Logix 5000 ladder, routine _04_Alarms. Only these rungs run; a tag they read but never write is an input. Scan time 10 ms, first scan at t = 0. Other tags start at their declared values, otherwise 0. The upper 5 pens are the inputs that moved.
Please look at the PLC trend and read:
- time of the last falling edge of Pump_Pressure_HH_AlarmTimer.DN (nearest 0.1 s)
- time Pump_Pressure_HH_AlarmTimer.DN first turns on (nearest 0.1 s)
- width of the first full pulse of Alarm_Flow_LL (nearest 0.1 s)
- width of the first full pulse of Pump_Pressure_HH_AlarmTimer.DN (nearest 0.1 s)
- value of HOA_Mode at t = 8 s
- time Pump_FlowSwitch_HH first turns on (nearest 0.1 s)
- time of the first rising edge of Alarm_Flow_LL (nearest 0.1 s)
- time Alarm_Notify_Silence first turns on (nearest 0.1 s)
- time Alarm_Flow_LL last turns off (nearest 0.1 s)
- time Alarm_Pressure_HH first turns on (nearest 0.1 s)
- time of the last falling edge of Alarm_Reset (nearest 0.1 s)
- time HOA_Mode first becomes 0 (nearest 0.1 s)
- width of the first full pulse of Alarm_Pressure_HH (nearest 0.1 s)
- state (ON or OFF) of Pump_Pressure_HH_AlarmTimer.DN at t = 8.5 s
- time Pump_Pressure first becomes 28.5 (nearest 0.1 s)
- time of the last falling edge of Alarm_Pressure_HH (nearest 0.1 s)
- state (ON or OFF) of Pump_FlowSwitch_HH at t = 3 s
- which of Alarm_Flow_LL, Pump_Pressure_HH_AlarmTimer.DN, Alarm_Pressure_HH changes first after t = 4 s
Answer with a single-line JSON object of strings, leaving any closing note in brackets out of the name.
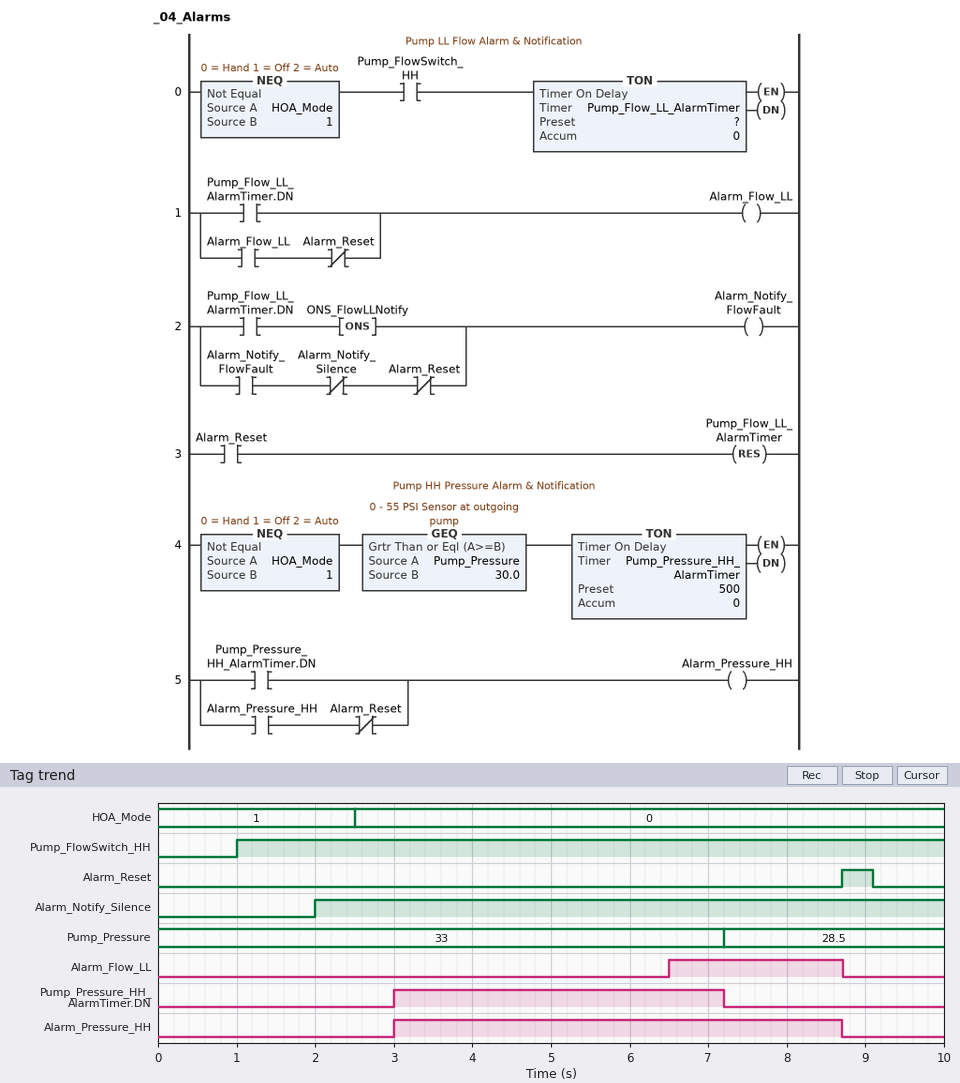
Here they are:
{"time of the last falling edge of Pump_Pressure_HH_AlarmTimer.DN": "7.2 s", "time Pump_Pressure_HH_AlarmTimer.DN first turns on": "3.0 s", "width of the first full pulse of Alarm_Flow_LL": "2.2 s", "width of the first full pulse of Pump_Pressure_HH_AlarmTimer.DN": "4.2 s", "value of HOA_Mode at t = 8 s": "0", "time Pump_FlowSwitch_HH first turns on": "1.0 s", "time of the first rising edge of Alarm_Flow_LL": "6.5 s", "time Alarm_Notify_Silence first turns on": "2.0 s", "time Alarm_Flow_LL last turns off": "8.7 s", "time Alarm_Pressure_HH first turns on": "3.0 s", "time of the last falling edge of Alarm_Reset": "9.1 s", "time HOA_Mode first becomes 0": "2.5 s", "width of the first full pulse of Alarm_Pressure_HH": "5.7 s", "state (ON or OFF) of Pump_Pressure_HH_AlarmTimer.DN at t = 8.5 s": "OFF", "time Pump_Pressure first becomes 28.5": "7.2 s", "time of the last falling edge of Alarm_Pressure_HH": "8.7 s", "state (ON or OFF) of Pump_FlowSwitch_HH at t = 3 s": "ON", "which of Alarm_Flow_LL, Pump_Pressure_HH_AlarmTimer.DN, Alarm_Pressure_HH changes first after t = 4 s": "Alarm_Flow_LL"}
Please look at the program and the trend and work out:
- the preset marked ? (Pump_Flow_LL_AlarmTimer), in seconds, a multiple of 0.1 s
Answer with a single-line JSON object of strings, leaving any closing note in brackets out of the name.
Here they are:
{"the preset marked ? (Pump_Flow_LL_AlarmTimer), in seconds, a multiple of 0.1 s": "4.0 s"}
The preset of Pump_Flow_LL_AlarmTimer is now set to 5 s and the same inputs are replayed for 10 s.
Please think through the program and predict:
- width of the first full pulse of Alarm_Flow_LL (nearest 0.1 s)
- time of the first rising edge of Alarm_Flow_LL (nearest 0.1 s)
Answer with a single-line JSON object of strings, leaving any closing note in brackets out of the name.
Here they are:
{"width of the first full pulse of Alarm_Flow_LL": "1.2 s", "time of the first rising edge of Alarm_Flow_LL": "7.5 s"}
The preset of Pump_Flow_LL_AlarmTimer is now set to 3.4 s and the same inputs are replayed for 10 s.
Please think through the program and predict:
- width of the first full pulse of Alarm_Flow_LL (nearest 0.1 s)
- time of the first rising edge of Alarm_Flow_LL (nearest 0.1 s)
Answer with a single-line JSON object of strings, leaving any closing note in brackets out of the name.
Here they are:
{"width of the first full pulse of Alarm_Flow_LL": "2.8 s", "time of the first rising edge of Alarm_Flow_LL": "5.9 s"}
